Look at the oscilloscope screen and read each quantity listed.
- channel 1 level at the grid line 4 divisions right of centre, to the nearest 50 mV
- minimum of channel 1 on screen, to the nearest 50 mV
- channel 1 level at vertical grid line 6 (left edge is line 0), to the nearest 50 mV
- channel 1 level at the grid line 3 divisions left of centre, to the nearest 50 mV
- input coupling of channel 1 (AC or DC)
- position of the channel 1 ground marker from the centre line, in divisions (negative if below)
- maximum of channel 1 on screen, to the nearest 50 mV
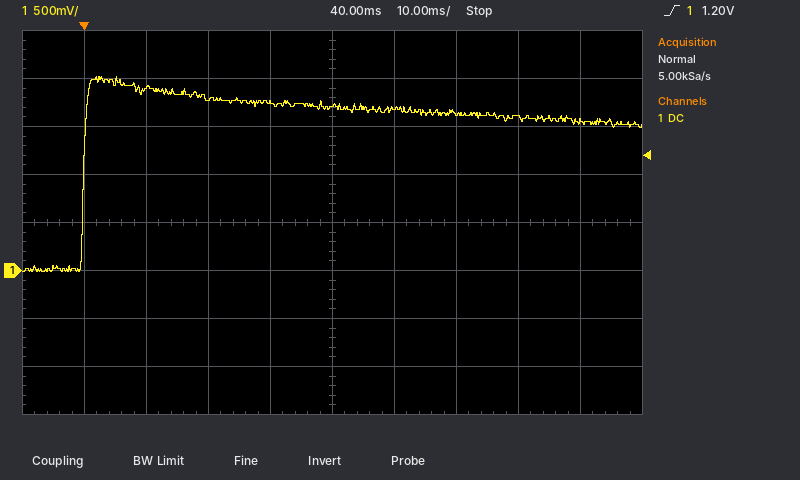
1.55 V
0 mV
1.70 V
1.90 V
DC
-1.0 div
2.00 V
